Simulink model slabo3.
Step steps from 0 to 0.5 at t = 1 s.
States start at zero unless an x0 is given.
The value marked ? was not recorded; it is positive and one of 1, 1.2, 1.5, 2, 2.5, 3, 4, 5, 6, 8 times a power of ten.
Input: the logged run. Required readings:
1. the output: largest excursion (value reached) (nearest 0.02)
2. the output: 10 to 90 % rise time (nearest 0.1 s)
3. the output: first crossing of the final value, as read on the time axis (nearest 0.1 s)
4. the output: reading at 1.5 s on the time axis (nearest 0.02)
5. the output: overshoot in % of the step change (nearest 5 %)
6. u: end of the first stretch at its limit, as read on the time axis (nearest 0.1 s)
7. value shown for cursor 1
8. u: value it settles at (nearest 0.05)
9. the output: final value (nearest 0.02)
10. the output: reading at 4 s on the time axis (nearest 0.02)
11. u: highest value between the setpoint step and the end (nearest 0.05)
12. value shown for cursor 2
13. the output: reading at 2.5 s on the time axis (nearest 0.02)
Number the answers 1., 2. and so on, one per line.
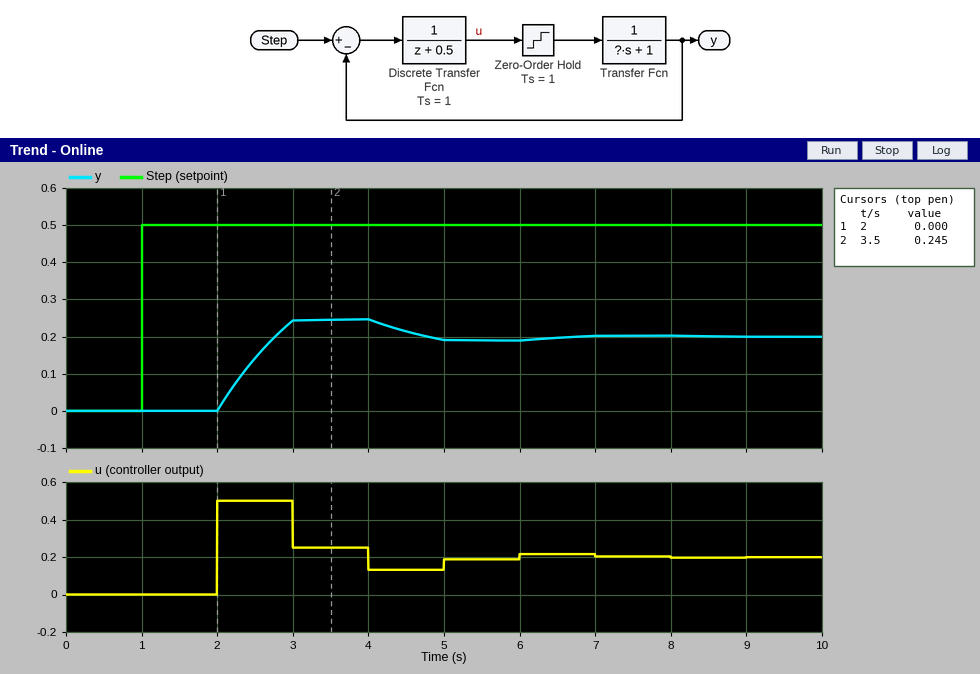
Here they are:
1. 0.24
2. 0.6 s
3. 2.8 s
4. 0.00
5. 25 %
6. 2.0 s
7. 0.000
8. 0.20
9. 0.20
10. 0.24
11. 0.50
12. 0.245
13. 0.14
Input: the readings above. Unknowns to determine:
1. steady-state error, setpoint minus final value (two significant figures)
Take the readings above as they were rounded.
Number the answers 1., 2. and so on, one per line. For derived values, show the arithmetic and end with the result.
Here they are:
1. 0.5 - 0.2 = 0.30
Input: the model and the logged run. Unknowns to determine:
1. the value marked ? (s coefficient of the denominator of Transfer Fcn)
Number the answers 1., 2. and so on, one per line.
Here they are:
1. 1.5
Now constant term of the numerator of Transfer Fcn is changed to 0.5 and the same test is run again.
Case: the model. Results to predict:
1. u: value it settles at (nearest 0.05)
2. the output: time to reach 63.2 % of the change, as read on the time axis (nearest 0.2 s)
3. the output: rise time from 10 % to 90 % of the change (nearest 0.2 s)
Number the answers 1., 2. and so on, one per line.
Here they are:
1. 0.25
2. 2.6 s
3. 0.8 s
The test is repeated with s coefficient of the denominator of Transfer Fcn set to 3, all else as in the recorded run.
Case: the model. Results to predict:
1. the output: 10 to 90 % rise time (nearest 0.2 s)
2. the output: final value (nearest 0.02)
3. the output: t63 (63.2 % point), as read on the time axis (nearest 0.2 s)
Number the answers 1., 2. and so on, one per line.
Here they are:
1. 2.2 s
2. 0.20
3. 2.8 s
